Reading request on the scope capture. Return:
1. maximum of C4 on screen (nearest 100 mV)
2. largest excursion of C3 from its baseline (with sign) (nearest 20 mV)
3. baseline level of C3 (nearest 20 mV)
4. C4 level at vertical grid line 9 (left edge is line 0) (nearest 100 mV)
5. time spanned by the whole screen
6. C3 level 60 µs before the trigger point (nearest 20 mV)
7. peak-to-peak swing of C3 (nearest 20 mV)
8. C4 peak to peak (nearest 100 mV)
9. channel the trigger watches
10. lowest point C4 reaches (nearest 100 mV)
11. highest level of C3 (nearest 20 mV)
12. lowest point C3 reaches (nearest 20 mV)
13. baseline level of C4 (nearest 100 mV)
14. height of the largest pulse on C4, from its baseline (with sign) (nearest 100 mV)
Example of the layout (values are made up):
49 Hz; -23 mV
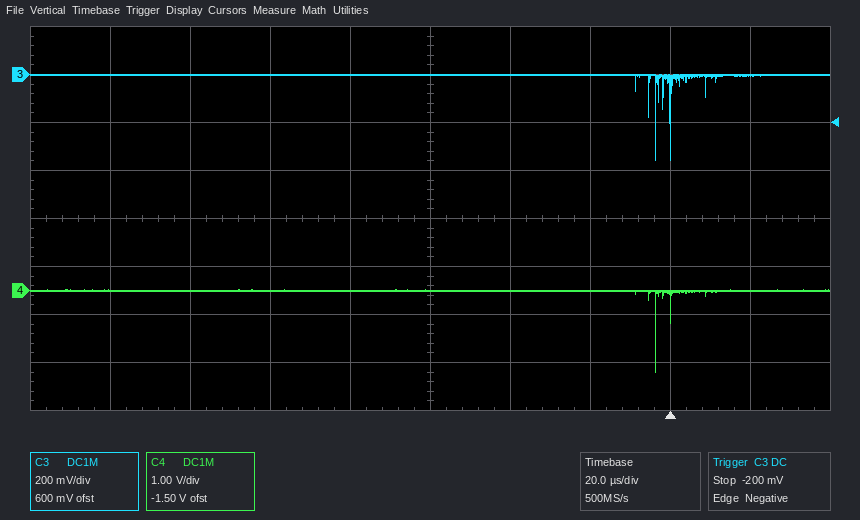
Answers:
0.0 V; -360 mV; 0 mV; 0.0 V; 200 µs; 0 mV; 360 mV; 1.7 V; C3; -1.7 V; 0 mV; -360 mV; 0.0 V; -1.7 V
